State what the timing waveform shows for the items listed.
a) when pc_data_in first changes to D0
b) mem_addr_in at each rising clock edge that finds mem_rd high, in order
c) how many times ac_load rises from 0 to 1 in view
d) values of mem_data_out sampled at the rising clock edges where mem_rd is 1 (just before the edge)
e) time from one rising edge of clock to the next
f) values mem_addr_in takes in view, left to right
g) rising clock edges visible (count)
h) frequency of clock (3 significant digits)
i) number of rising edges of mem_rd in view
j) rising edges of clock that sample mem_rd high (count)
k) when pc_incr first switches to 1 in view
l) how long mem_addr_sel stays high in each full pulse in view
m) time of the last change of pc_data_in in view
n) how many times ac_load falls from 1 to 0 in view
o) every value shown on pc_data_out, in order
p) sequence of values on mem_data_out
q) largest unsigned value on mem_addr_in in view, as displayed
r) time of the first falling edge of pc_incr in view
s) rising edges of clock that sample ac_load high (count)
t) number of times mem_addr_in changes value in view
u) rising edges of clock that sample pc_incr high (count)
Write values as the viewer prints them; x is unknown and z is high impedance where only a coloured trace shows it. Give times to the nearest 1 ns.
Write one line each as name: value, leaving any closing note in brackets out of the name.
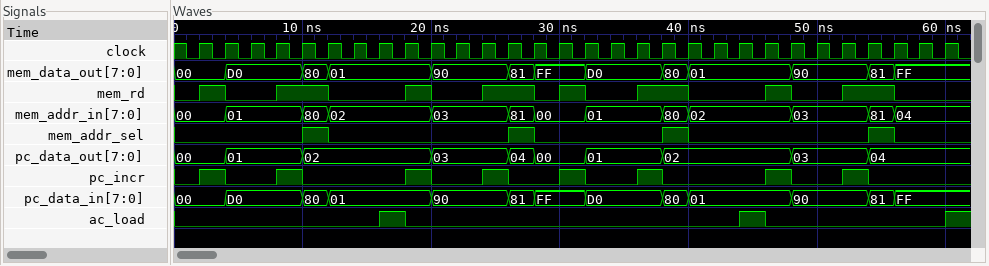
when pc_data_in first changes to D0: 4 ns
mem_addr_in at each rising clock edge that finds mem_rd high, in order: 00, 01, 80, 02, 03, 81, 00, 01, 80, 02, 03, 81
how many times ac_load rises from 0 to 1 in view: 3
values of mem_data_out sampled at the rising clock edges where mem_rd is 1: 00, D0, 80, 01, 90, 81, FF, D0, 80, 01, 90, 81
time from one rising edge of clock to the next: 2 ns
values mem_addr_in takes in view, left to right: 00, 01, 80, 02, 03, 81, 00, 01, 80, 02, 03, 81, 04
rising clock edges visible: 30
frequency of clock: 500 MHz
number of rising edges of mem_rd in view: 8
rising edges of clock that sample mem_rd high: 12
when pc_incr first switches to 1 in view: 2 ns
how long mem_addr_sel stays high in each full pulse in view: 2 ns, 2 ns, 2 ns, 2 ns
time of the last change of pc_data_in in view: 56 ns
how many times ac_load falls from 1 to 0 in view: 2
every value shown on pc_data_out, in order: 00, 01, 02, 03, 04, 00, 01, 02, 03, 04
sequence of values on mem_data_out: 00, D0, 80, 01, 90, 81, FF, D0, 80, 01, 90, 81, FF
largest unsigned value on mem_addr_in in view, as displayed: 81
time of the first falling edge of pc_incr in view: 4 ns
rising edges of clock that sample ac_load high: 2
number of times mem_addr_in changes value in view: 12
rising edges of clock that sample pc_incr high: 8
